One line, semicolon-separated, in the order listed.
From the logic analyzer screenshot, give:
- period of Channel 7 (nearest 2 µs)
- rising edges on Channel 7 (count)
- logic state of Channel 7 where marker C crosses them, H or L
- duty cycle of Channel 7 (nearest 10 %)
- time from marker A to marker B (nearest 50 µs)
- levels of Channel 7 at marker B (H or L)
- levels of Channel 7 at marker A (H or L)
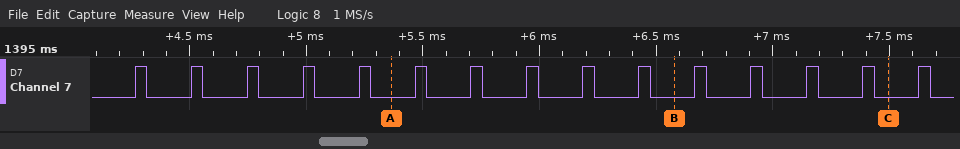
240 µs; 15; Channel 7=L; 20 %; 1200 µs; Channel 7=L; Channel 7=L
